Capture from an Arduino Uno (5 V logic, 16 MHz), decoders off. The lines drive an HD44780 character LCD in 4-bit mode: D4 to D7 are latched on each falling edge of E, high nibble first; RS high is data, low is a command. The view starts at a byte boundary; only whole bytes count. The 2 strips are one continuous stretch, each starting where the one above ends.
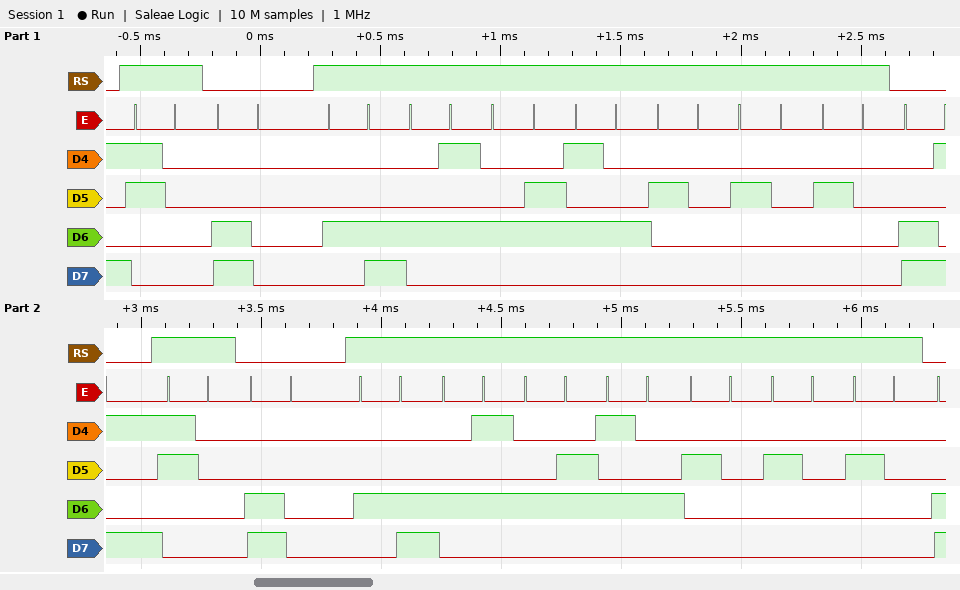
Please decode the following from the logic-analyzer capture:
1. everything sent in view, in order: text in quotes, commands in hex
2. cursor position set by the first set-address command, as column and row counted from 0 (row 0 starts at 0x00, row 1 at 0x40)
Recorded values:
"0" 0xC0 "LEFT   " 0xC9 "0" 0xC0 "LEFT   "
column 0, row 1
